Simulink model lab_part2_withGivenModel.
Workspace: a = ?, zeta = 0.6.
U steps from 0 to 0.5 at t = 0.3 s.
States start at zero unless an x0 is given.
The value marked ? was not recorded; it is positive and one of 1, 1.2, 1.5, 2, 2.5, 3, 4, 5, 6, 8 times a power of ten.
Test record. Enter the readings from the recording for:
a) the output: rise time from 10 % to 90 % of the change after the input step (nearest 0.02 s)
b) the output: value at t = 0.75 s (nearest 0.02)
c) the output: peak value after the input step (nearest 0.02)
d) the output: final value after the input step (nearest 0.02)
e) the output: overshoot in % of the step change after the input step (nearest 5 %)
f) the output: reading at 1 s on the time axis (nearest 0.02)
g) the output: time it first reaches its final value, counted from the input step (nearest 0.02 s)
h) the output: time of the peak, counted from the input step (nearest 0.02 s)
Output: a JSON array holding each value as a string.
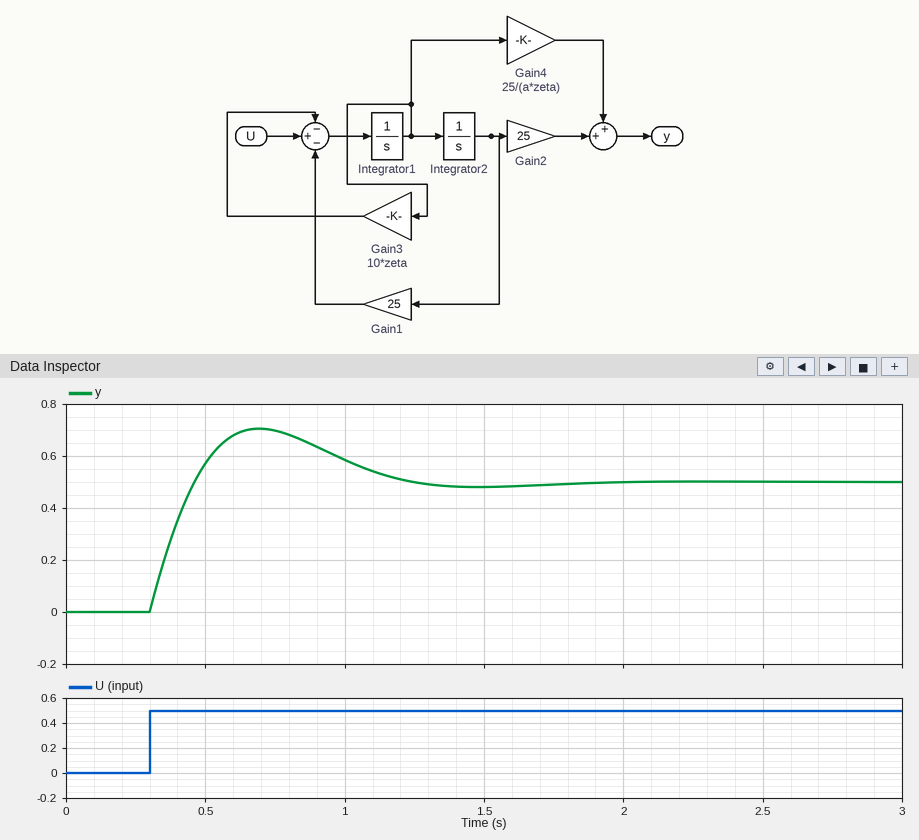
["0.12 s", "0.70", "0.70", "0.50", "40 %", "0.58", "0.16 s", "0.40 s"]
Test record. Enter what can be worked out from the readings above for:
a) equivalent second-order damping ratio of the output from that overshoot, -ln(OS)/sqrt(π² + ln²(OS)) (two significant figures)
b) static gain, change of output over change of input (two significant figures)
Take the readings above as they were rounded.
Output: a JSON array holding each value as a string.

["0.28", "1.0"]
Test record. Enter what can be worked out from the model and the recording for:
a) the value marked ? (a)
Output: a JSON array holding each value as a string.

["5"]
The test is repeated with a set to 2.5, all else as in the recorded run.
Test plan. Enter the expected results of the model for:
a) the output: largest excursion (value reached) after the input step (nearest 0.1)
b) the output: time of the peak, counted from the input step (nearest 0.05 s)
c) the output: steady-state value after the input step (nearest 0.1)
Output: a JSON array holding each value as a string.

["1.1", "0.30 s", "0.5"]
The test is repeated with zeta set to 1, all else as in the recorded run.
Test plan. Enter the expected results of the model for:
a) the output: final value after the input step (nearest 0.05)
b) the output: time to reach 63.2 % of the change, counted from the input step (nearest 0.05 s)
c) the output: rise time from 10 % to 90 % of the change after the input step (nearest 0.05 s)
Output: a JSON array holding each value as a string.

["0.50", "0.20 s", "0.45 s"]
